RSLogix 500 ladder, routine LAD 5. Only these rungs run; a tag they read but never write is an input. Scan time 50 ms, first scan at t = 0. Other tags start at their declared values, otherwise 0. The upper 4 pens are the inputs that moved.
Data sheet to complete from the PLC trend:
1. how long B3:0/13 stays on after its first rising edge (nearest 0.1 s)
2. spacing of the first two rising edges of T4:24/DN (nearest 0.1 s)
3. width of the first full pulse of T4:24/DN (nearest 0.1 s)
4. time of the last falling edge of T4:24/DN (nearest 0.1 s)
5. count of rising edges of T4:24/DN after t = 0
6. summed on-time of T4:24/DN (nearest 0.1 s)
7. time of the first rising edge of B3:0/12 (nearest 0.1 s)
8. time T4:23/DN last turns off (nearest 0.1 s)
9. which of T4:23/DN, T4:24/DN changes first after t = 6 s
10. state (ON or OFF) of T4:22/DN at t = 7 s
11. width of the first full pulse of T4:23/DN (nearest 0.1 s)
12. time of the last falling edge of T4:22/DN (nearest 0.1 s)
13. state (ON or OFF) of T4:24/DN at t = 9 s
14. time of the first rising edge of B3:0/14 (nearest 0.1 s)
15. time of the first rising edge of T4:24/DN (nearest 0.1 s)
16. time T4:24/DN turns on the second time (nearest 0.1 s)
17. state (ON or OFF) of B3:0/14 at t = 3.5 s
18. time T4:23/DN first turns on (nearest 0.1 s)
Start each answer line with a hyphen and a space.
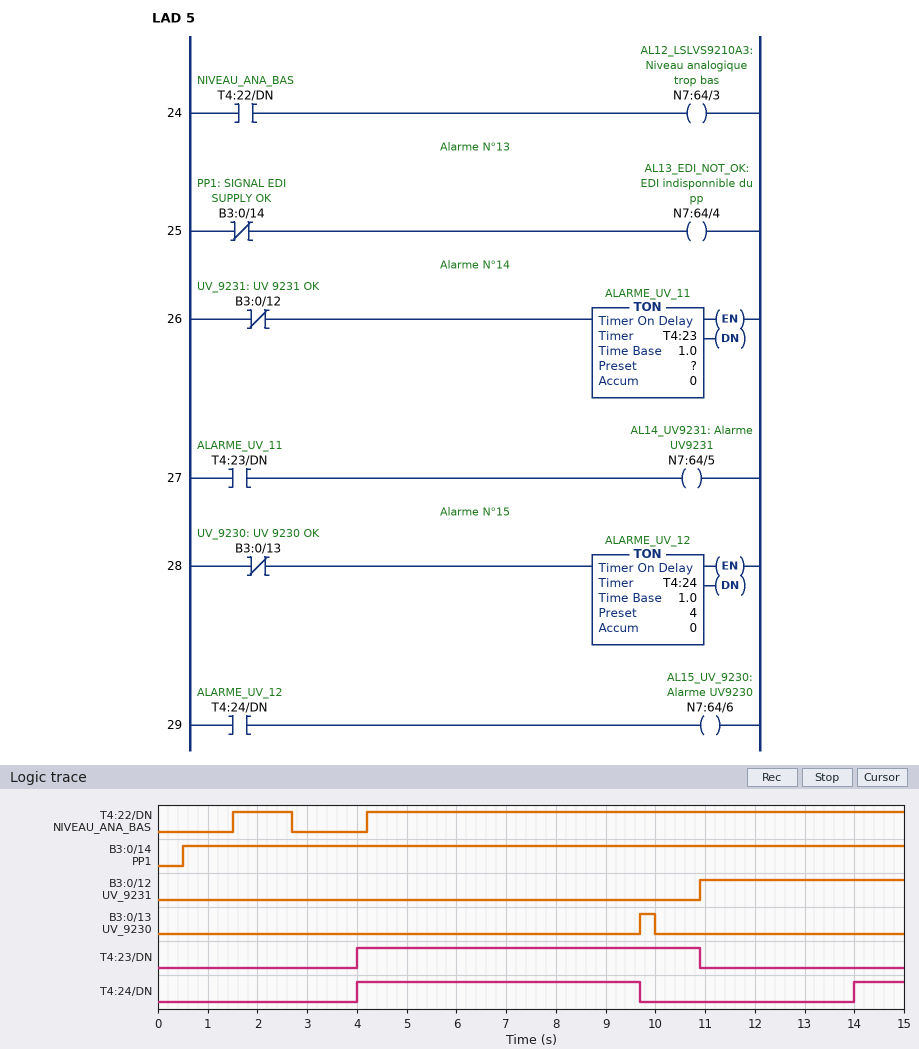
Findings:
- 0.3 s
- 10.0 s
- 5.7 s
- 9.7 s
- 2
- 6.7 s
- 10.9 s
- 10.9 s
- T4:24/DN
- ON
- 6.9 s
- 2.7 s
- ON
- 0.5 s
- 4.0 s
- 14.0 s
- ON
- 4.0 s
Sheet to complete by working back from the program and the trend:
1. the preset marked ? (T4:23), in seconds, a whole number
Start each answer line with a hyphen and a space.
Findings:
- 4 s
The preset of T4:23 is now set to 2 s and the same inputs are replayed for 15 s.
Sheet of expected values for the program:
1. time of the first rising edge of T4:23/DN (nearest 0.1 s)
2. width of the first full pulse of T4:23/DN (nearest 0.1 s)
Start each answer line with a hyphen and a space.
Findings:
- 2.0 s
- 8.9 s
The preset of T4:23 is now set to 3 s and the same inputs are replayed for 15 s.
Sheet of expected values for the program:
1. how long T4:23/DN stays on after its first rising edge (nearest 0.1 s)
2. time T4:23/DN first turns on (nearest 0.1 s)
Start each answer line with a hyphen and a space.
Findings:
- 7.9 s
- 3.0 s
